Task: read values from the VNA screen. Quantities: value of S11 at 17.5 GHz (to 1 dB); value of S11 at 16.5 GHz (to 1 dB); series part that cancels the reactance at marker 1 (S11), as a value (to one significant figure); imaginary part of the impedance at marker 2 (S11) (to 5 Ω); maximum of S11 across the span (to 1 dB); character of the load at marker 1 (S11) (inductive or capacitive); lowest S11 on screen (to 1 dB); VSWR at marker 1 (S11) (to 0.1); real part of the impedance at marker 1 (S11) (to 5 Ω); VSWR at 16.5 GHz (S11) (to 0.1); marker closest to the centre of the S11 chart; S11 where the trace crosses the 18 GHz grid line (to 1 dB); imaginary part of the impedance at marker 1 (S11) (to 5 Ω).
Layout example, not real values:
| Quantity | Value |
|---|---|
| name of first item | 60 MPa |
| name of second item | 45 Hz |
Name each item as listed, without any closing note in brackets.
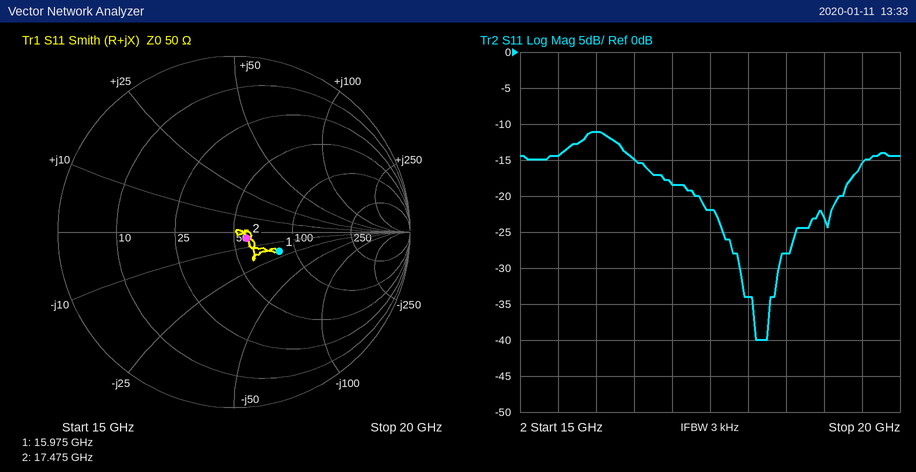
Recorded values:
| Quantity | Value |
|---|---|
| value of S11 at 17.5 GHz | -22 dB |
| value of S11 at 16.5 GHz | -15 dB |
| series part that cancels the reactance at marker 1 (S11), as a value | 200 pH |
| imaginary part of the impedance at marker 2 (S11) | -5 Ω |
| maximum of S11 across the span | -11 dB |
| character of the load at marker 1 (S11) | capacitive |
| lowest S11 on screen | -40 dB |
| VSWR at marker 1 (S11) | 1.8 |
| real part of the impedance at marker 1 (S11) | 80 Ω |
| VSWR at 16.5 GHz (S11) | 1.4 |
| marker closest to the centre of the S11 chart | marker 2 |
| S11 where the trace crosses the 18 GHz grid line | -34 dB |
| imaginary part of the impedance at marker 1 (S11) | -20 Ω |
